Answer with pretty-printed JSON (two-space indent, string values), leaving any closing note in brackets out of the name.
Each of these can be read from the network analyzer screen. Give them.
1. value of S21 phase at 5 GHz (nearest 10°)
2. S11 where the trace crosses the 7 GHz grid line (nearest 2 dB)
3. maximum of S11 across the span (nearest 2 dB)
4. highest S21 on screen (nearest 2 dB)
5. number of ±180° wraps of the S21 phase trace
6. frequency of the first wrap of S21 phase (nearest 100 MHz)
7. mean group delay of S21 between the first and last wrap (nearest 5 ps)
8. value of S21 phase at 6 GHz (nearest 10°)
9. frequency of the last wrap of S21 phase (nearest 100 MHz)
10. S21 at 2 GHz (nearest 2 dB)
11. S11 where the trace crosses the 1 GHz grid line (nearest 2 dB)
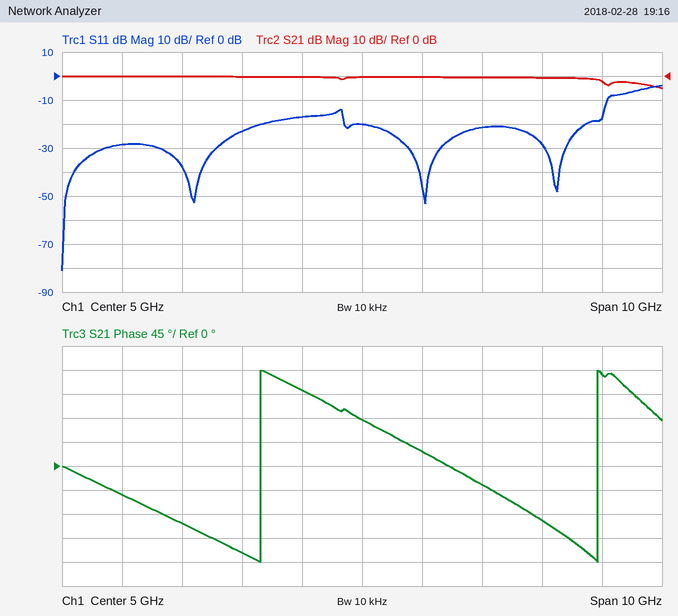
{
  "value of S21 phase at 5 GHz": "90°",
  "S11 where the trace crosses the 7 GHz grid line": "-22 dB",
  "maximum of S11 across the span": "-4 dB",
  "highest S21 on screen": "0 dB",
  "number of ±180° wraps of the S21 phase trace": "2",
  "frequency of the first wrap of S21 phase": "3.3 GHz",
  "mean group delay of S21 between the first and last wrap": "180 ps",
  "value of S21 phase at 6 GHz": "30°",
  "frequency of the last wrap of S21 phase": "8.9 GHz",
  "S21 at 2 GHz": "0 dB",
  "S11 where the trace crosses the 1 GHz grid line": "-28 dB"
}
